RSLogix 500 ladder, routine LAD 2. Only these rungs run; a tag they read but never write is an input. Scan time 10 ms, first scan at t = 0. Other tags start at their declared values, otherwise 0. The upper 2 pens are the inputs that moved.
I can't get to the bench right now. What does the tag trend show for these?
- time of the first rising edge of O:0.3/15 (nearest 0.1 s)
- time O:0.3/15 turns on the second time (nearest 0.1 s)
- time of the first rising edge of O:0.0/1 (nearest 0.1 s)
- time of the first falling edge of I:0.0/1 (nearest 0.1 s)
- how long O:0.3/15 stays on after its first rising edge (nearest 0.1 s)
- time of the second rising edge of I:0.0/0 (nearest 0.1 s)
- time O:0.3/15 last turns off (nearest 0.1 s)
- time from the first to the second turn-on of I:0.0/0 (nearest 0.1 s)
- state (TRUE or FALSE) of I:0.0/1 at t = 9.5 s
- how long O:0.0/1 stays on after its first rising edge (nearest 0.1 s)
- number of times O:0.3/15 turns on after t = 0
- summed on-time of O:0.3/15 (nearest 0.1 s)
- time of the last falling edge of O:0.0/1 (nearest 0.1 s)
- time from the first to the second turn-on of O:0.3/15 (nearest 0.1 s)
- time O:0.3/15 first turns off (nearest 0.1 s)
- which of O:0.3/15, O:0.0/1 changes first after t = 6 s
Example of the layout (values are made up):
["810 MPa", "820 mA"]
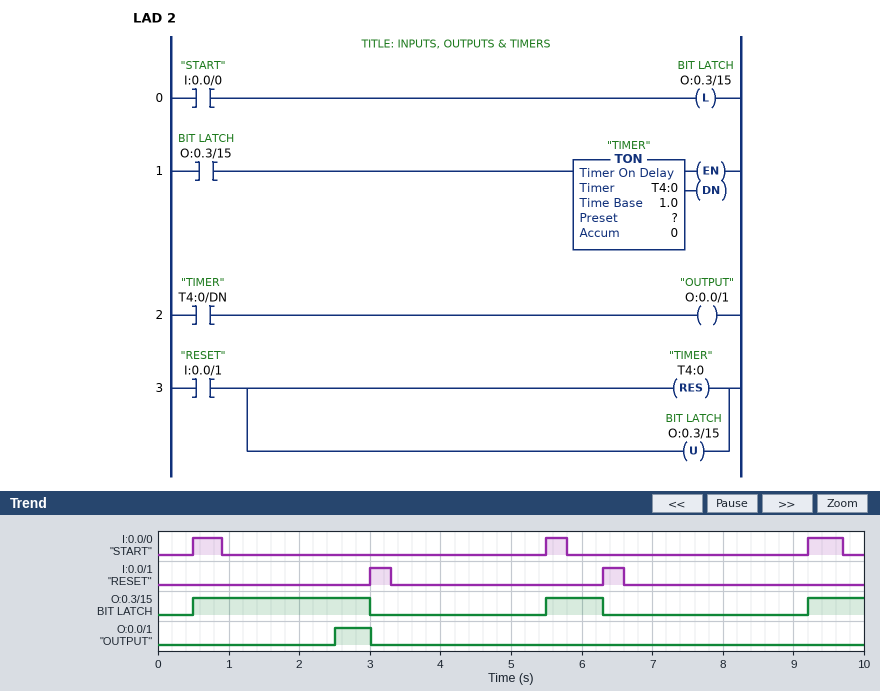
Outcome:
["0.5 s", "5.5 s", "2.5 s", "3.3 s", "2.5 s", "5.5 s", "6.3 s", "5.0 s", "FALSE", "0.5 s", "3", "4.1 s", "3.0 s", "5.0 s", "3.0 s", "O:0.3/15"]
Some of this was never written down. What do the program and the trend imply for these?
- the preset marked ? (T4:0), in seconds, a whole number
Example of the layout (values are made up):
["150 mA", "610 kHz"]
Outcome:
["2 s"]
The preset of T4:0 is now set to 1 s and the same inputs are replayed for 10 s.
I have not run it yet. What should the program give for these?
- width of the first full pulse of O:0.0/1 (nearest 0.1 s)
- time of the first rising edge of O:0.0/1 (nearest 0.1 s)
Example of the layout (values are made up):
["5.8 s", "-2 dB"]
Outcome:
["1.5 s", "1.5 s"]
